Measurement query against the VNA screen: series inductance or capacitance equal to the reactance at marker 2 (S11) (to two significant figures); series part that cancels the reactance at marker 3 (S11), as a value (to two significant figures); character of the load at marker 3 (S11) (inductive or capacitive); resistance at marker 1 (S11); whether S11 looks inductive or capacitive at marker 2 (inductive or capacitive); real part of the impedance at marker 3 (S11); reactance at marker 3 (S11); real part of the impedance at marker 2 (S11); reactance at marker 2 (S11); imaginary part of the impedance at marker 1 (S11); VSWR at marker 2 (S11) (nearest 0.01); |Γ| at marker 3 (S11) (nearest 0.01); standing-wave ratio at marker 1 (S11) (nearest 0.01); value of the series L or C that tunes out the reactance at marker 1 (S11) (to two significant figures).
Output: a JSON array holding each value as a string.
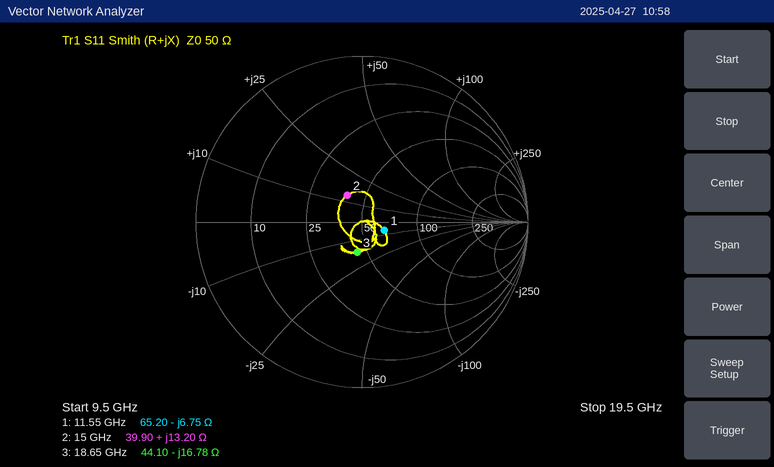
["140 pH", "140 pH", "capacitive", "65.20 Ω", "inductive", "44.10 Ω", "-16.78 Ω", "39.90 Ω", "+13.20 Ω", "-6.75 Ω", "1.45", "0.19", "1.34", "93 pH"]
